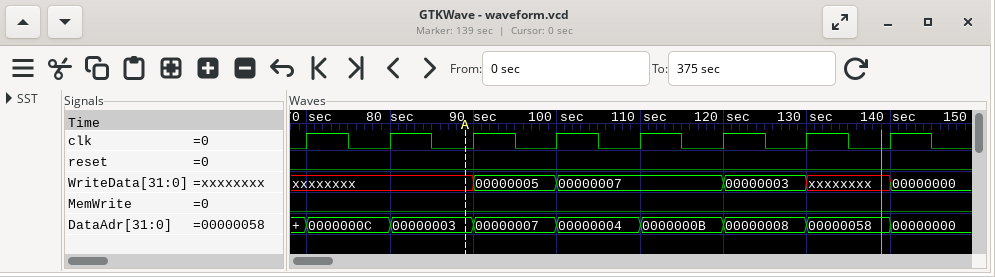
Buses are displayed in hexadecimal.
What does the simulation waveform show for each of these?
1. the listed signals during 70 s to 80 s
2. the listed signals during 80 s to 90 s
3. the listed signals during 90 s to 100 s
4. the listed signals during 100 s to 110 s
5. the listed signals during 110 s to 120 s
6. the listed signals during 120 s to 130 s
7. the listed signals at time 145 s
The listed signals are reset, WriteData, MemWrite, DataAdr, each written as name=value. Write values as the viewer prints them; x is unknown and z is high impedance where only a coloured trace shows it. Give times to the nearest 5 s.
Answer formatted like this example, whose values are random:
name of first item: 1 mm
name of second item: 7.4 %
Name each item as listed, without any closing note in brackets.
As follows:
the listed signals during 70 s to 80 s: reset=0, WriteData=xxxxxxxx, MemWrite=0, DataAdr=0000000C
the listed signals during 80 s to 90 s: reset=0, WriteData=xxxxxxxx, MemWrite=0, DataAdr=00000003
the listed signals during 90 s to 100 s: reset=0, WriteData=00000005, MemWrite=0, DataAdr=00000007
the listed signals during 100 s to 110 s: reset=0, WriteData=00000007, MemWrite=0, DataAdr=00000004
the listed signals during 110 s to 120 s: reset=0, WriteData=00000007, MemWrite=0, DataAdr=0000000B
the listed signals during 120 s to 130 s: reset=0, WriteData=00000003, MemWrite=0, DataAdr=00000008
the listed signals at time 145 s: reset=0, WriteData=00000000, MemWrite=0, DataAdr=00000000
